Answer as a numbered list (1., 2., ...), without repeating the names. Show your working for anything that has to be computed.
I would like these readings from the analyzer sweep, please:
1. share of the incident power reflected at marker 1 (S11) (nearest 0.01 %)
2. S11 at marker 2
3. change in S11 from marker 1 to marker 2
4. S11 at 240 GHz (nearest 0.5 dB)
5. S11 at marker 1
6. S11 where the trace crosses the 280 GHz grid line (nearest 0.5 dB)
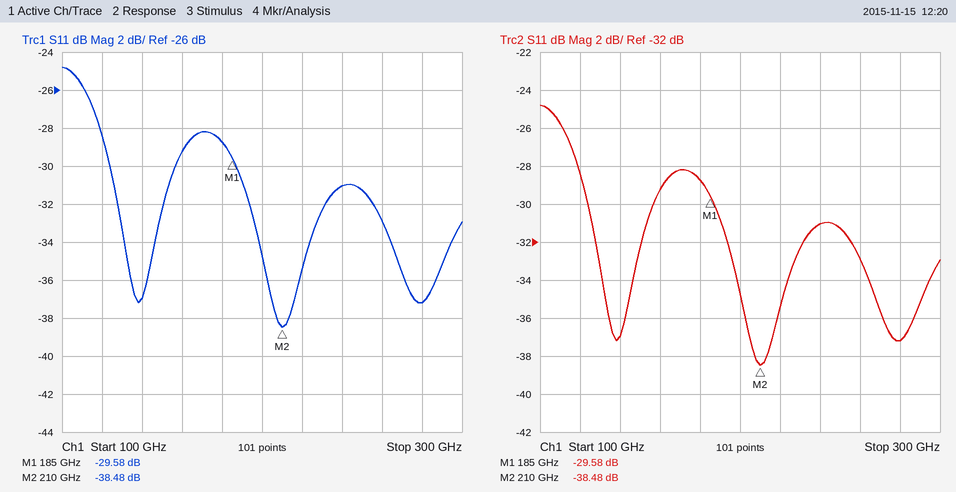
1. 10^(-29.58/10) ≈ 0.11 %
2. -38.48 dB
3. -38.48 − (-29.58) = -8.90 dB
4. -31.0 dB
5. -29.58 dB
6. -37.0 dB
